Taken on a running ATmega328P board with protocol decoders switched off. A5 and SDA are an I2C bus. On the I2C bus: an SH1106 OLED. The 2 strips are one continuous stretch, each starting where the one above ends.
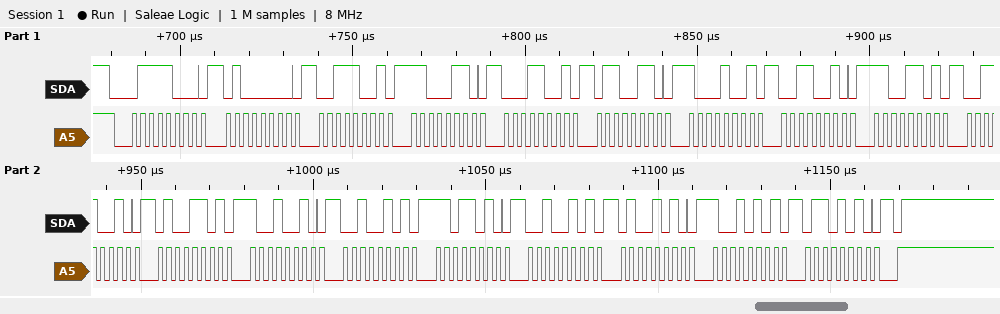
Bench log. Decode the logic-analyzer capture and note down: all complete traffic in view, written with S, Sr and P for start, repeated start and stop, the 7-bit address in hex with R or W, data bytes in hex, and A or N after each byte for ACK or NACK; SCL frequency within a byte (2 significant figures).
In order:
S 3CW A 40 A 39 A C6 A 19 A 66 A 89 A 32 A CD A 32 A 4D A 92 A 25 A DA A 25 A 4A A 95 A 6A A P
400 kHz
